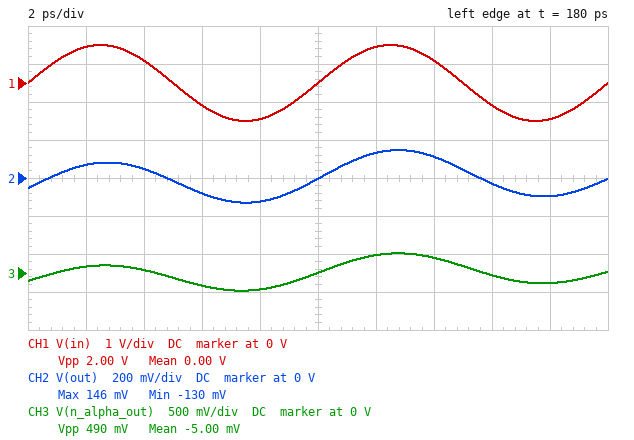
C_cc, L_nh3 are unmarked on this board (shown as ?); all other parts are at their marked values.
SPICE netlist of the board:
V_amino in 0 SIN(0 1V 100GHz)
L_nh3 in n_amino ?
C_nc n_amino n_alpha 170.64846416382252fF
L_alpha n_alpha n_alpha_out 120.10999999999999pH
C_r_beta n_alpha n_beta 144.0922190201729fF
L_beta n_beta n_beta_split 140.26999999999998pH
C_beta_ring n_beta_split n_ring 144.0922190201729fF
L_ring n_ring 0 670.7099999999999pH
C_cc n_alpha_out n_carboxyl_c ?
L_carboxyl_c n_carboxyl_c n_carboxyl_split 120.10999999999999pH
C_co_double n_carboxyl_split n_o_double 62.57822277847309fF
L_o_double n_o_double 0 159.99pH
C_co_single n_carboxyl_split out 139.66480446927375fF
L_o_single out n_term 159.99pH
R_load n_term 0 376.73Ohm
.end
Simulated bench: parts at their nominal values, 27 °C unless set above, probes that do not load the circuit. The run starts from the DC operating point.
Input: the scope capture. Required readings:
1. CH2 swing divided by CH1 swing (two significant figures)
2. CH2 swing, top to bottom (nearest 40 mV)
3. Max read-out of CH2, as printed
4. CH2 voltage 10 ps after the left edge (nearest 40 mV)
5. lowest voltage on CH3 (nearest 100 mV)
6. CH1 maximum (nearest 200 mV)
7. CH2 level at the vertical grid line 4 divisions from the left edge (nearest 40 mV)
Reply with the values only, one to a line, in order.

0.14
280 mV
146 mV
0 V
-200 mV
1.0 V
-120 mV
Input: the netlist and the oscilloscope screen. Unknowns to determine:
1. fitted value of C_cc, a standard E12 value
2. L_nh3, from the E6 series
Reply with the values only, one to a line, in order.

56 fF
470 pH
